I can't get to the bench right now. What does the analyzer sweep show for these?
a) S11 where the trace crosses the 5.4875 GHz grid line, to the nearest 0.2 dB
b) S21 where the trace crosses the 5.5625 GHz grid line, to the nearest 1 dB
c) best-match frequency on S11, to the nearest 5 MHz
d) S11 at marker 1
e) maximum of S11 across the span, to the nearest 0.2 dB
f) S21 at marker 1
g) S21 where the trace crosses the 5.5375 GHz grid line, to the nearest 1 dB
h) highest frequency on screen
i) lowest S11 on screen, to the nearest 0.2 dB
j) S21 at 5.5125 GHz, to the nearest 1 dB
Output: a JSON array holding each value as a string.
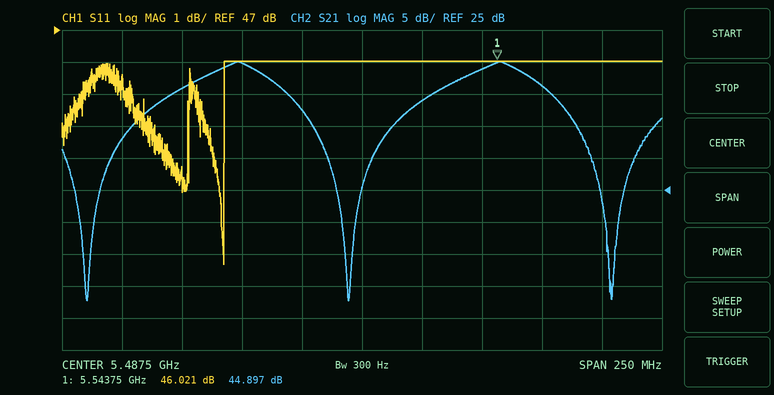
["46.0 dB", "41 dB", "5.430 GHz", "46.021 dB", "46.0 dB", "44.897 dB", "44 dB", "5.6125 GHz", "39.6 dB", "39 dB"]
